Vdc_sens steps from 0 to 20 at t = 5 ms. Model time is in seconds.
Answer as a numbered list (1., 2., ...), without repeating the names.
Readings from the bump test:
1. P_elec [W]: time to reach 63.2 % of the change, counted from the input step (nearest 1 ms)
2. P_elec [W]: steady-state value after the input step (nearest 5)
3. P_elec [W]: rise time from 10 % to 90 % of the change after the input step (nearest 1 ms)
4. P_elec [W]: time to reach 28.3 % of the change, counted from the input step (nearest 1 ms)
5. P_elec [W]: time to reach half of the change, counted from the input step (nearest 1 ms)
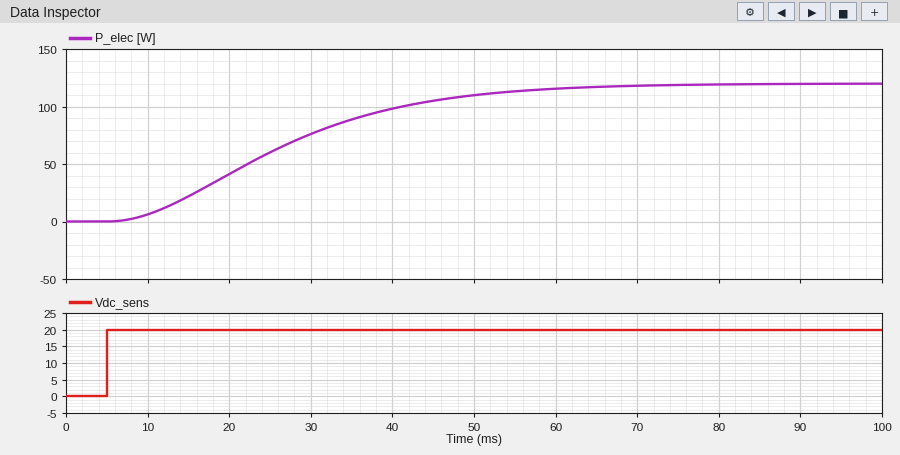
1. 25 ms
2. 120
3. 36 ms
4. 13 ms
5. 20 ms
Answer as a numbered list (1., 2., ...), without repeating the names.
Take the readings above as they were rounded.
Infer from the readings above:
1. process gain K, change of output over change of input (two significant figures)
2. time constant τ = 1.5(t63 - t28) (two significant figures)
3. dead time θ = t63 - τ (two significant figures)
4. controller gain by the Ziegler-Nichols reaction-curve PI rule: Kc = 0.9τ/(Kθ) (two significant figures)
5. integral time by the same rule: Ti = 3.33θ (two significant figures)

1. 6.0
2. 18 ms
3. 7.0 ms
4. 0.39
5. 23 ms
